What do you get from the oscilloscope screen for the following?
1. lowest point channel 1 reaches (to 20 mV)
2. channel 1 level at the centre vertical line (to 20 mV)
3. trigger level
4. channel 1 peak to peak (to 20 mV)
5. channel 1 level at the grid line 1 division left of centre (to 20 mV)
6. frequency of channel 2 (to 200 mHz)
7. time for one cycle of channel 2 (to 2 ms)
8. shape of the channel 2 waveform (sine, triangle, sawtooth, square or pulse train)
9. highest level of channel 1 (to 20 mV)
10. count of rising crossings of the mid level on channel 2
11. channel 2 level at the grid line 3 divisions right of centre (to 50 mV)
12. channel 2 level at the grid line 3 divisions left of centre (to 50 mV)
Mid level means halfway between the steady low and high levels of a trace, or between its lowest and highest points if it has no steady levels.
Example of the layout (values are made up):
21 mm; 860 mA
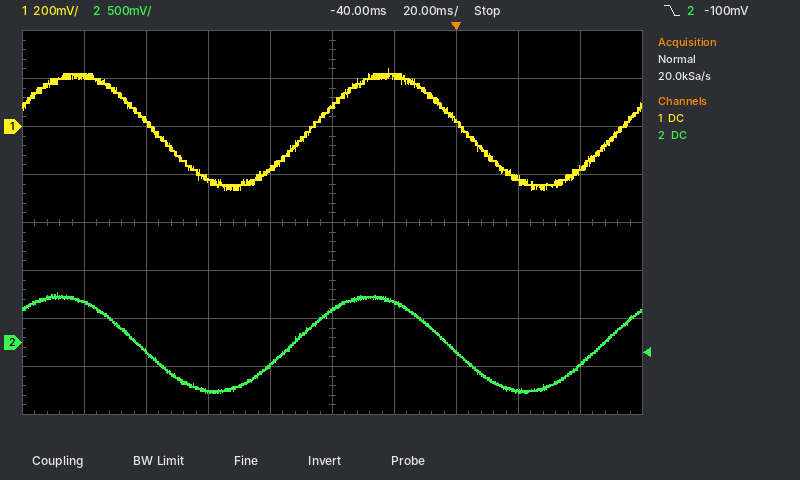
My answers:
-260 mV; 80 mV; -100 mV; 500 mV; -180 mV; 10.0 Hz; 100 ms; sine; 240 mV; 2; -500 mV; -100 mV
